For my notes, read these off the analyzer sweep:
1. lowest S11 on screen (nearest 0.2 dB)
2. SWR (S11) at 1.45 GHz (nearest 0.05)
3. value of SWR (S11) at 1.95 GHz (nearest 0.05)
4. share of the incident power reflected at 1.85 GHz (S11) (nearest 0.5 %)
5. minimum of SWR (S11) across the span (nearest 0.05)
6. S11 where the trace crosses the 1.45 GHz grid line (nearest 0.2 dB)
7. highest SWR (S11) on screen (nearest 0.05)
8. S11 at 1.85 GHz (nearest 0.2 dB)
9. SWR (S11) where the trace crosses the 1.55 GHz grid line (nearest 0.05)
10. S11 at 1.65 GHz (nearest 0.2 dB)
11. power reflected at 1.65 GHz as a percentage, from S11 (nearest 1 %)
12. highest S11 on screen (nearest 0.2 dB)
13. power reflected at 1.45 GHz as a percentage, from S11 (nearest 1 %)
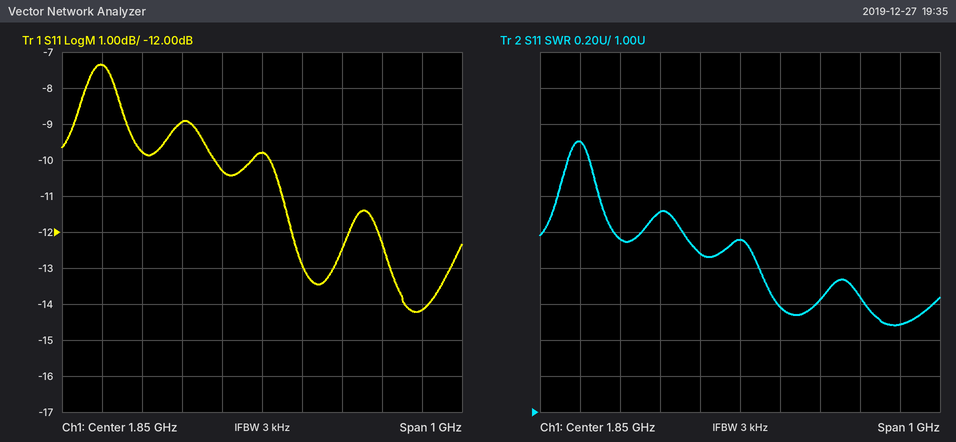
-14.2 dB
2.50
1.60
10.5 %
1.50
-7.4 dB
2.50
-9.8 dB
1.95
-9.0 dB
13 %
-7.4 dB
18 %
